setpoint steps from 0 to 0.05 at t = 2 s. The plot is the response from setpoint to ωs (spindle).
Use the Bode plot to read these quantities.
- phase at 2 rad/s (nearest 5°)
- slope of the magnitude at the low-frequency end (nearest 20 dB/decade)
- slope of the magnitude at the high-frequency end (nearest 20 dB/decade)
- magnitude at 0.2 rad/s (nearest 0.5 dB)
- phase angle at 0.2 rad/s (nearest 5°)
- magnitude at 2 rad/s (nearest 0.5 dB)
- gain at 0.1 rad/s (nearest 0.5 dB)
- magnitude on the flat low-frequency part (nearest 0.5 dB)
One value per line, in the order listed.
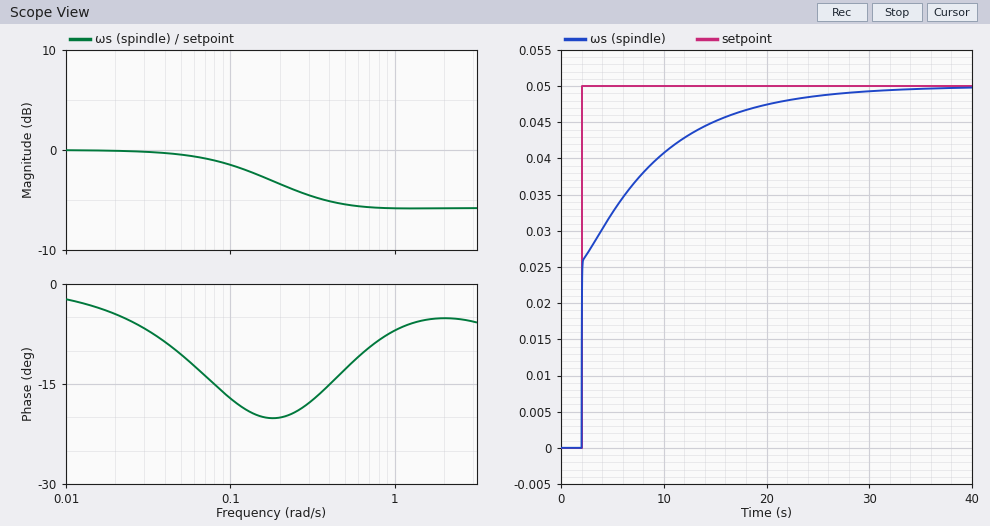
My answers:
-5°
0 dB/decade
0 dB/decade
-3.5 dB
-20°
-6.0 dB
-1.5 dB
0.0 dB
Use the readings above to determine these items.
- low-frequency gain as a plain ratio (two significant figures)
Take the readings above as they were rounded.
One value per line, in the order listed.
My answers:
1.0
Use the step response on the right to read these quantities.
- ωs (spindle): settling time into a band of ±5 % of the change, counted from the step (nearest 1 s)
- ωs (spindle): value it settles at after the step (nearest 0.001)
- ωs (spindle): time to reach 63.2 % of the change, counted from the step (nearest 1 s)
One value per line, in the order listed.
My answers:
18 s
0.050
3 s
